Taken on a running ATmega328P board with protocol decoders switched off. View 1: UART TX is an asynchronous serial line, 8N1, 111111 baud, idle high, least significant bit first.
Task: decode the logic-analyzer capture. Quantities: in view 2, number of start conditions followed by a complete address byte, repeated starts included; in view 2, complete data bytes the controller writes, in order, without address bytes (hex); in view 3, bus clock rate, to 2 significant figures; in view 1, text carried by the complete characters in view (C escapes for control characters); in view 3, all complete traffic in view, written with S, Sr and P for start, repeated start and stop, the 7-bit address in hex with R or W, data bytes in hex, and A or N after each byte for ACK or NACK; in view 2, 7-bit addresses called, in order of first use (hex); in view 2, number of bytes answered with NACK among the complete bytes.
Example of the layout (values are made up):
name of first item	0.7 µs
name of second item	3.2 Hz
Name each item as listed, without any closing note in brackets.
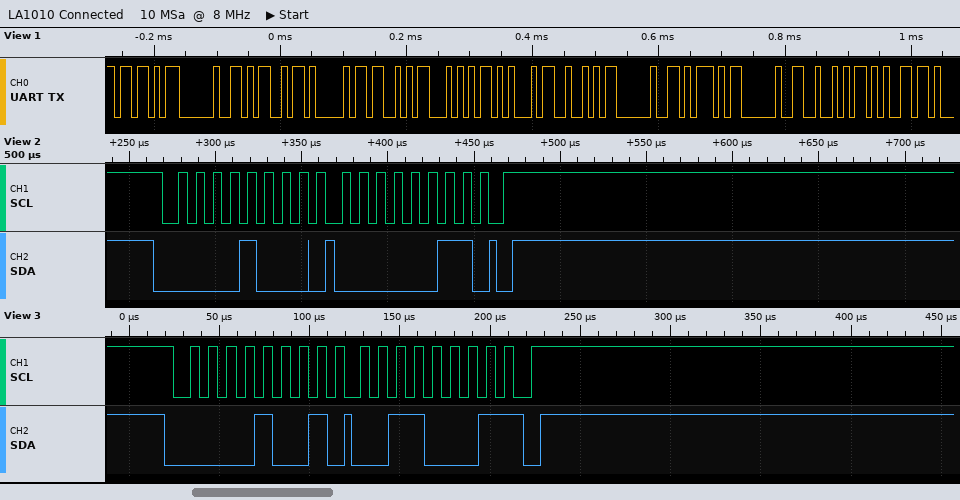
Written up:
in view 2, number of start conditions followed by a complete address byte, repeated starts included	1
in view 2, complete data bytes the controller writes, in order, without address bytes	03
in view 3, bus clock rate, to 2 significant figures	100 kHz
in view 1, text carried by the complete characters in view	"[ MASTER ] Re"
in view 3, all complete traffic in view, written with S, Sr and P for start, repeated start and stop, the 7-bit address in hex with R or W, data bytes in hex, and A or N after each byte for ACK or NACK	S 04R A 31 N P
in view 2, 7-bit addresses called, in order of first use	0x04
in view 2, number of bytes answered with NACK among the complete bytes	0
